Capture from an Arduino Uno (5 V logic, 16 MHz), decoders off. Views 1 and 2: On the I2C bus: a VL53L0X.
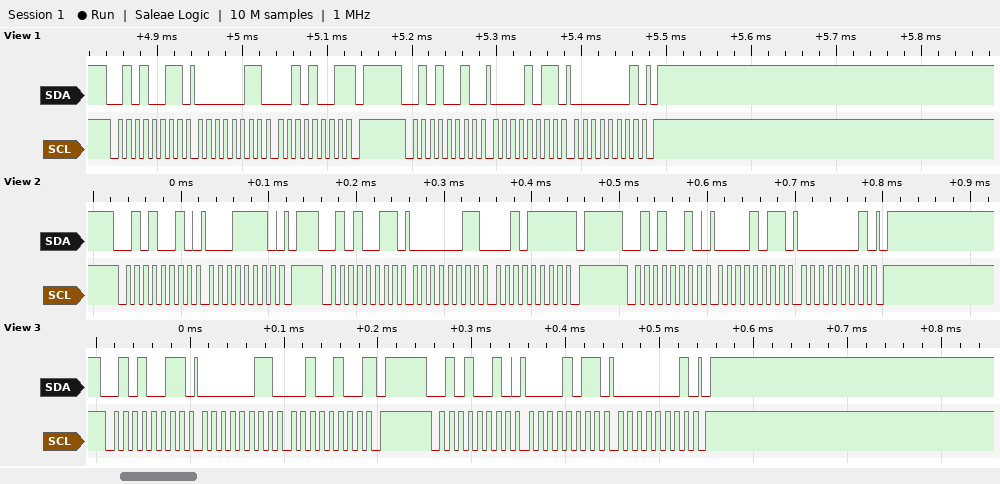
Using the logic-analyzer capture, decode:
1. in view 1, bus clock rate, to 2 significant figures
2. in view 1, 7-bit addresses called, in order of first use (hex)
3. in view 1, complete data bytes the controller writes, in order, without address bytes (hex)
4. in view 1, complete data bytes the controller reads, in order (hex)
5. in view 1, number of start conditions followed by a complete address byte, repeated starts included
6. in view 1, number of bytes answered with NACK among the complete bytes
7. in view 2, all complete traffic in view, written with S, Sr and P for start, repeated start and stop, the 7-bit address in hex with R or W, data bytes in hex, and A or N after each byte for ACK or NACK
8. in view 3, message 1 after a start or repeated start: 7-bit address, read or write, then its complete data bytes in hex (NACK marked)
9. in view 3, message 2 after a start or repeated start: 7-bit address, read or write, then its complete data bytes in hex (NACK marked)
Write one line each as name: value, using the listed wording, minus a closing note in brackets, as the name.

in view 1, bus clock rate, to 2 significant figures: 100 kHz
in view 1, 7-bit addresses called, in order of first use: 0x29
in view 1, complete data bytes the controller writes, in order, without address bytes: 0B 01
in view 1, complete data bytes the controller reads, in order: 03 29
in view 1, number of start conditions followed by a complete address byte, repeated starts included: 2
in view 1, number of bytes answered with NACK among the complete bytes: 1
in view 2, all complete traffic in view, written with S, Sr and P for start, repeated start and stop, the 7-bit address in hex with R or W, data bytes in hex, and A or N after each byte for ACK or NACK: S 29W A 1E A P S 29R A 03 A 2F N P S 29W A 0B A 01 A P
in view 3, message 1 after a start or repeated start: 7-bit address, read or write, then its complete data bytes in hex: 0x29 read: 03 24 NACK
in view 3, message 2 after a start or repeated start: 7-bit address, read or write, then its complete data bytes in hex: 0x29 write: 0B 01
